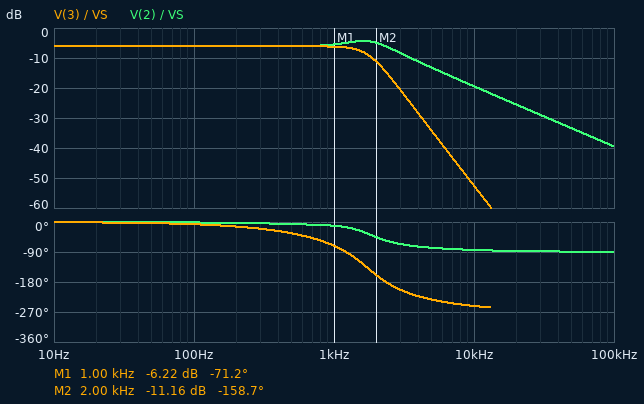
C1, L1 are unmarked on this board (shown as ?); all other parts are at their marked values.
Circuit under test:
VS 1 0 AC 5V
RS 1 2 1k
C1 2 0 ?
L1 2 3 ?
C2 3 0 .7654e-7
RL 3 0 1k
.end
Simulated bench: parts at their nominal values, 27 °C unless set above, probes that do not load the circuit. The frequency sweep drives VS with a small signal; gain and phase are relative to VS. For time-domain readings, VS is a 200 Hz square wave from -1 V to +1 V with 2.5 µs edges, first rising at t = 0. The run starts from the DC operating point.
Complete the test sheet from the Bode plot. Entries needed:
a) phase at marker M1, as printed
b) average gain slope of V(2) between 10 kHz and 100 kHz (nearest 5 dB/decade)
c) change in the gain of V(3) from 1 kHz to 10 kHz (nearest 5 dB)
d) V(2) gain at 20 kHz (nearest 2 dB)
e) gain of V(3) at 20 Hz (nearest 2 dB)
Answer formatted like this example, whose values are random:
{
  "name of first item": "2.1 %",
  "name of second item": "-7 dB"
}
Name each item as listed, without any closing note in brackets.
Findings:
{
  "phase at marker M1, as printed": "-71.2 deg",
  "average gain slope of V(2) between 10 kHz and 100 kHz": "-20 dB/decade",
  "change in the gain of V(3) from 1 kHz to 10 kHz": "-45 dB",
  "V(2) gain at 20 kHz": "-26 dB",
  "gain of V(3) at 20 Hz": "-6 dB"
}
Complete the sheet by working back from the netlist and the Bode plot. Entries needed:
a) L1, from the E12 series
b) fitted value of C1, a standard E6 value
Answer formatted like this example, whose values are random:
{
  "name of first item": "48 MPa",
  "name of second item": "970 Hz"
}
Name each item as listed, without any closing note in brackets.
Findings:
{
  "L1, from the E12 series": "150 mH",
  "fitted value of C1, a standard E6 value": "150 nF"
}
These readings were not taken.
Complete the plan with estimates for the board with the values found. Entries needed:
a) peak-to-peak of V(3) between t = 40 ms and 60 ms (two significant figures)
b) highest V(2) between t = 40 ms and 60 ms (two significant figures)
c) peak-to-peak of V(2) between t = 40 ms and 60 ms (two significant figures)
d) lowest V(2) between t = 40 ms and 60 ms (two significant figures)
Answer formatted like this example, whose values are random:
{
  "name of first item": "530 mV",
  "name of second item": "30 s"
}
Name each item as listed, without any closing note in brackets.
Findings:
{
  "peak-to-peak of V(3) between t = 40 ms and 60 ms": "1.2 V",
  "highest V(2) between t = 40 ms and 60 ms": "640 mV",
  "peak-to-peak of V(2) between t = 40 ms and 60 ms": "1.3 V",
  "lowest V(2) between t = 40 ms and 60 ms": "-640 mV"
}
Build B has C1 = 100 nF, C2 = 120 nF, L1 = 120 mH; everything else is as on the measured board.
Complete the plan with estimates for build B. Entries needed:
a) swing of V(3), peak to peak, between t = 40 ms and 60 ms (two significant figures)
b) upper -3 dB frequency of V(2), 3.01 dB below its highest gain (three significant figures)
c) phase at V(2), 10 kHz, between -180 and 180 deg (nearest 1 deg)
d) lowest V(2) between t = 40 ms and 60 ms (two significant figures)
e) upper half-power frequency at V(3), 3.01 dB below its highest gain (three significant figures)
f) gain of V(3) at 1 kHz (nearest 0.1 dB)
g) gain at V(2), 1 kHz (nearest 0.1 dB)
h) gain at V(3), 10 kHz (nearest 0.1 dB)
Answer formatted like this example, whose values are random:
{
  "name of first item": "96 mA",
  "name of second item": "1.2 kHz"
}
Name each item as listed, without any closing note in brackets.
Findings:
{
  "swing of V(3), peak to peak, between t = 40 ms and 60 ms": "1.2 V",
  "upper -3 dB frequency of V(2), 3.01 dB below its highest gain": "3.20 kHz",
  "phase at V(2), 10 kHz, between -180 and 180 deg": "-81 deg",
  "lowest V(2) between t = 40 ms and 60 ms": "-670 mV",
  "upper half-power frequency at V(3), 3.01 dB below its highest gain": "2.09 kHz",
  "gain of V(3) at 1 kHz": "-6.1 dB",
  "gain at V(2), 1 kHz": "-7.3 dB",
  "gain at V(3), 10 kHz": "-50.9 dB"
}
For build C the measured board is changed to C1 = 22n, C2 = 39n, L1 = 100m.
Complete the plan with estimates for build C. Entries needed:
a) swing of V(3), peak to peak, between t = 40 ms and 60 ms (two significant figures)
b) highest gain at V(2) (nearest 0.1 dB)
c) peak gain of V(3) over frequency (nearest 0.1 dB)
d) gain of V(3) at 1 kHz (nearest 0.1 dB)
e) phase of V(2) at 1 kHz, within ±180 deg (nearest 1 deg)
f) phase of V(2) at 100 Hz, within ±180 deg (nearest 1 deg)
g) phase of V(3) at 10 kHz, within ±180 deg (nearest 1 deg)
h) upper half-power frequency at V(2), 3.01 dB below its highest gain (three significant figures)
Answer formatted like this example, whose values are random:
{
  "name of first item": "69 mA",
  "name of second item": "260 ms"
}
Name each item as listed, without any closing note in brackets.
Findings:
{
  "swing of V(3), peak to peak, between t = 40 ms and 60 ms": "1.1 V",
  "highest gain at V(2)": "-0.8 dB",
  "peak gain of V(3) over frequency": "-6.0 dB",
  "gain of V(3) at 1 kHz": "-6.1 dB",
  "phase of V(2) at 1 kHz, within ±180 deg": "7 deg",
  "phase of V(2) at 100 Hz, within ±180 deg": "1 deg",
  "phase of V(3) at 10 kHz, within ±180 deg": "153 deg",
  "upper half-power frequency at V(2), 3.01 dB below its highest gain": "9.82 kHz"
}
